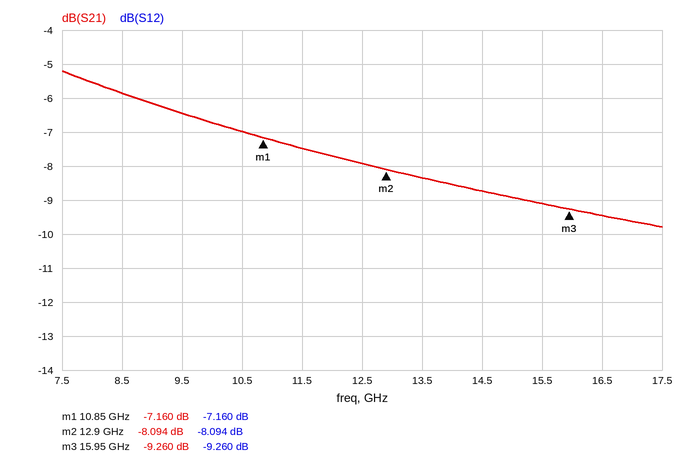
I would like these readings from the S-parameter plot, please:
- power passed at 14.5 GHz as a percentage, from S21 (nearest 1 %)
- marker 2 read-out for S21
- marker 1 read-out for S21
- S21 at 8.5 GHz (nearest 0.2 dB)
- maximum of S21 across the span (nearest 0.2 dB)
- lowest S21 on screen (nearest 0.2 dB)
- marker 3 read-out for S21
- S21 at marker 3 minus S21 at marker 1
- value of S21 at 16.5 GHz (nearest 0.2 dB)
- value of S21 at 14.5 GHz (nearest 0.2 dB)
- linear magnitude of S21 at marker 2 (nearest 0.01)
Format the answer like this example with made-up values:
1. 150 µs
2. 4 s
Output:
1. 13 %
2. -8.094 dB
3. -7.160 dB
4. -5.8 dB
5. -5.2 dB
6. -9.8 dB
7. -9.260 dB
8. -2.100 dB
9. -9.4 dB
10. -8.8 dB
11. 0.39
